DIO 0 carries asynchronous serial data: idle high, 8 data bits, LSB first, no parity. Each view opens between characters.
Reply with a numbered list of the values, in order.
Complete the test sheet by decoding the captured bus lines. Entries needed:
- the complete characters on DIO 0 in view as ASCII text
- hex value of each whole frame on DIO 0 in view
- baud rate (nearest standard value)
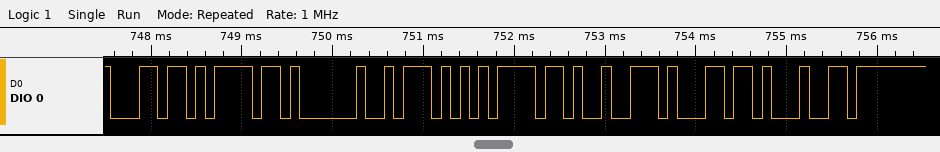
1. "lo World"
2. 6C, 6F, 20, 57, 6F, 72, 6C, 64
3. 9600 baud
